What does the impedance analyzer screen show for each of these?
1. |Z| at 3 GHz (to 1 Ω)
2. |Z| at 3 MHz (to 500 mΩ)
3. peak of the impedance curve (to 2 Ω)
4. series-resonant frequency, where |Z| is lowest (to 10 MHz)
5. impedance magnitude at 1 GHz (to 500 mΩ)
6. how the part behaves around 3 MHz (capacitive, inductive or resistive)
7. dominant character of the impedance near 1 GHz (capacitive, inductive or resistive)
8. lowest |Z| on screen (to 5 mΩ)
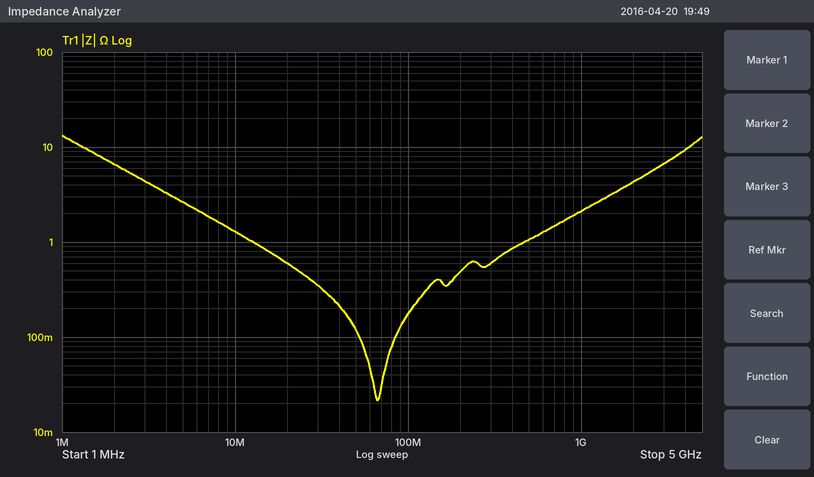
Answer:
7 Ω
4.5 Ω
14 Ω
70 MHz
2.0 Ω
capacitive
inductive
20 mΩ
